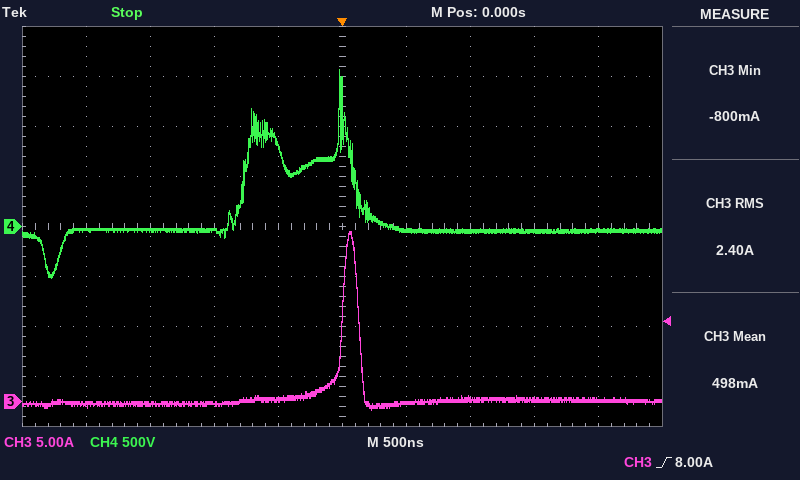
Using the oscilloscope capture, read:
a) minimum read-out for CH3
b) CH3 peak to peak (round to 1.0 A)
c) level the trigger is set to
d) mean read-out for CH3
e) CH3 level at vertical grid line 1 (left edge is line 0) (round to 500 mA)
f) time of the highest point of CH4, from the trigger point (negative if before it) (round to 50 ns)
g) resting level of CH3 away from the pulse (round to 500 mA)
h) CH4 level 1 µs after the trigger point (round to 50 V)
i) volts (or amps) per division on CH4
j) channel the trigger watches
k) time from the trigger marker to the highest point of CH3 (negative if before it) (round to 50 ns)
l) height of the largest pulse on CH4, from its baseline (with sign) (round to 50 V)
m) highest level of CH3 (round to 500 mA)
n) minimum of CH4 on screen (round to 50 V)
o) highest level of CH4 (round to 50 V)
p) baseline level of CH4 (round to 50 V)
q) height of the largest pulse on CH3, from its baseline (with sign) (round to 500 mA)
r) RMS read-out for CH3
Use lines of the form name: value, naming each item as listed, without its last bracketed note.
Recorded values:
minimum read-out for CH3: -800 mA
CH3 peak to peak: 18.0 A
level the trigger is set to: 8.00 A
mean read-out for CH3: 498 mA
CH3 level at vertical grid line 1 (left edge is line 0): -500 mA
time of the highest point of CH4, from the trigger point (negative if before it): 0 ns
resting level of CH3 away from the pulse: 0.0 A
CH4 level 1 µs after the trigger point: -50 V
volts (or amps) per division on CH4: 500 V
channel the trigger watches: CH3
time from the trigger marker to the highest point of CH3 (negative if before it): +50 ns
height of the largest pulse on CH4, from its baseline (with sign): +1.60 kV
highest level of CH3: 17.0 A
minimum of CH4 on screen: -500 V
highest level of CH4: 1.55 kV
baseline level of CH4: -50 V
height of the largest pulse on CH3, from its baseline (with sign): +17.0 A
RMS read-out for CH3: 2.40 A
